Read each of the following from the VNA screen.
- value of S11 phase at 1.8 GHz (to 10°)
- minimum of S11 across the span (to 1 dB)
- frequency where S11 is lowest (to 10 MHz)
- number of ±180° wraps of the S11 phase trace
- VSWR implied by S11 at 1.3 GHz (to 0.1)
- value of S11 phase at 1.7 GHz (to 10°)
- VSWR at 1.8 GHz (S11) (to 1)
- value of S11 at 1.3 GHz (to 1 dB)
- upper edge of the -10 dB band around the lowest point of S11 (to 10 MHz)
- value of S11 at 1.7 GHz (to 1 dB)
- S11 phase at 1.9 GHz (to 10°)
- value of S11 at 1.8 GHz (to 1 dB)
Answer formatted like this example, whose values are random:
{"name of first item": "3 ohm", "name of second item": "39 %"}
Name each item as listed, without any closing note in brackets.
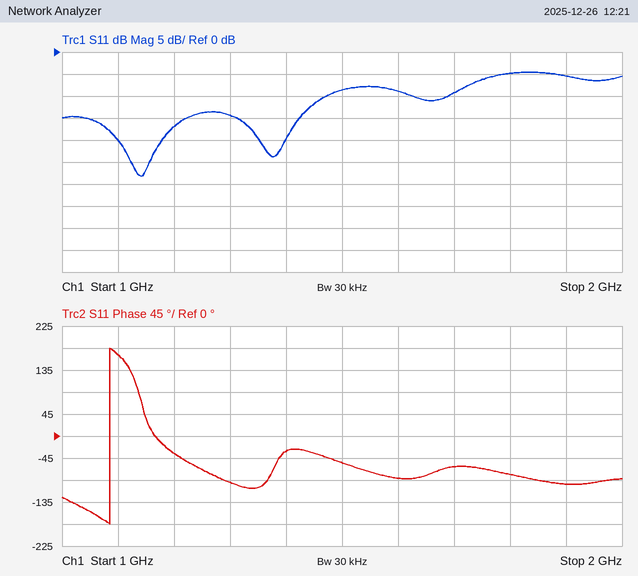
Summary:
{"value of S11 phase at 1.8 GHz": "-80°", "minimum of S11 across the span": "-28 dB", "frequency where S11 is lowest": "1.14 GHz", "number of ±180° wraps of the S11 phase trace": "1", "VSWR implied by S11 at 1.3 GHz": "1.5", "value of S11 phase at 1.7 GHz": "-60°", "VSWR at 1.8 GHz (S11)": "4", "value of S11 at 1.3 GHz": "-14 dB", "upper edge of the -10 dB band around the lowest point of S11": "1.47 GHz", "value of S11 at 1.7 GHz": "-9 dB", "S11 phase at 1.9 GHz": "-100°", "value of S11 at 1.8 GHz": "-5 dB"}
